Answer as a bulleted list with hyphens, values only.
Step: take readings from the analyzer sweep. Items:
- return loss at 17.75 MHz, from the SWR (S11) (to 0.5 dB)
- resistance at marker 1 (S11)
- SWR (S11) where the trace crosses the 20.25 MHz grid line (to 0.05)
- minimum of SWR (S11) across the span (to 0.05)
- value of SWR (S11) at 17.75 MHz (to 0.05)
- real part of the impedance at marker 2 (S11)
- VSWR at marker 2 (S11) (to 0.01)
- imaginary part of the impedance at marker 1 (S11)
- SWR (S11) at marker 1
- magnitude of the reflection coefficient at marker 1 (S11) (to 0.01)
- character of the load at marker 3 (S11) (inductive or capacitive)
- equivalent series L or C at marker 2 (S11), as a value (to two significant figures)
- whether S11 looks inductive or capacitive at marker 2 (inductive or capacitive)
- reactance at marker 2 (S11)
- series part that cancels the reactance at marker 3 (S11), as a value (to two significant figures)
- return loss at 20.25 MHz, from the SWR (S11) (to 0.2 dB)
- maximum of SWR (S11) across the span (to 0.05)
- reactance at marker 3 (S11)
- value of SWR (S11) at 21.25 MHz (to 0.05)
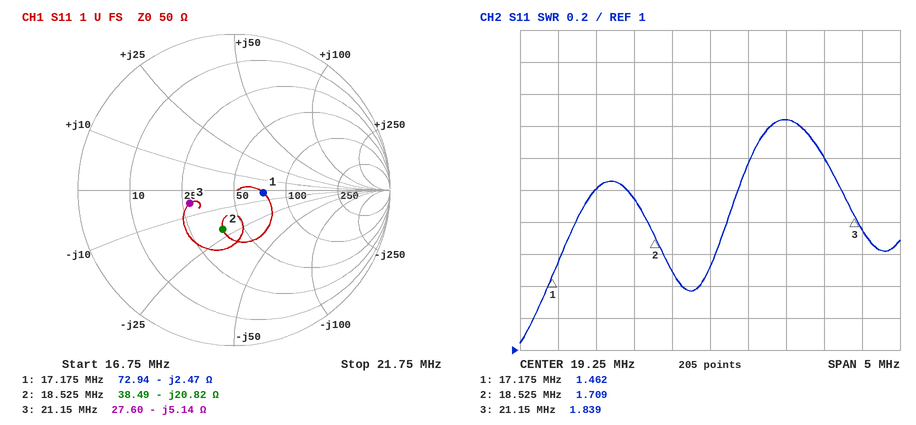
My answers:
- 9.5 dB
- 72.94 Ω
- 2.45
- 1.05
- 2.00
- 38.49 Ω
- 1.71
- -2.47 Ω
- 1.462
- 0.19
- capacitive
- 410 pF
- capacitive
- -20.82 Ω
- 39 nH
- 7.6 dB
- 2.45
- -5.14 Ω
- 1.75
